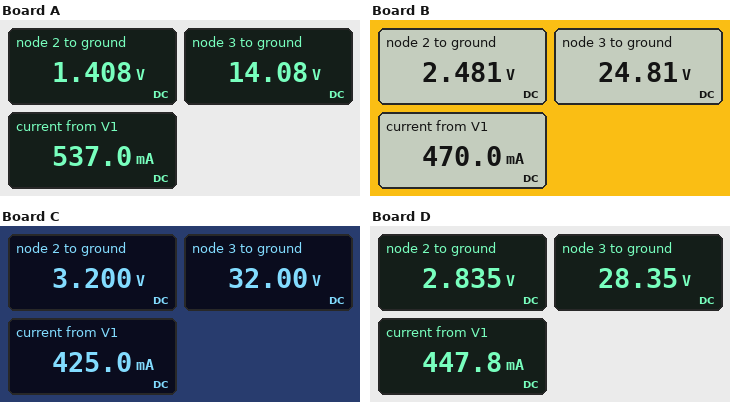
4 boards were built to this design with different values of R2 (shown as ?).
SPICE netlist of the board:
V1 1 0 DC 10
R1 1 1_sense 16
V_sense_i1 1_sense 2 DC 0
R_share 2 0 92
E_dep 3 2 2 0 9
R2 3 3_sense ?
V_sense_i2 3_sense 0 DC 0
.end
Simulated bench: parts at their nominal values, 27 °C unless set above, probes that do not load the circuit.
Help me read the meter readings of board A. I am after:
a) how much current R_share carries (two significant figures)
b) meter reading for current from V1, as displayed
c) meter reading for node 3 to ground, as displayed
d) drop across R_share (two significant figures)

15 mA
537.0 mA
14.08 V
1.4 V
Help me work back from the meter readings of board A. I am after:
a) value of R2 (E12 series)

27 Ω
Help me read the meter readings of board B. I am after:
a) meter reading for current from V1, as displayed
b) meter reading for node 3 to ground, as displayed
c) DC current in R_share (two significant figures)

470.0 mA
24.81 V
27 mA
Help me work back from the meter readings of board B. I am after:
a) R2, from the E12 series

56 Ω
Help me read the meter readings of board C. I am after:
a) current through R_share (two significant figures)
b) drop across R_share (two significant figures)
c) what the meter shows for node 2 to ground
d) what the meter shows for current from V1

35 mA
3.2 V
3.200 V
425.0 mA
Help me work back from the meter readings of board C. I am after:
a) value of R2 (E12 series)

82 Ω
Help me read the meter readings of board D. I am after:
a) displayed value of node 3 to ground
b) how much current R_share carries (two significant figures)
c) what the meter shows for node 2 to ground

28.35 V
31 mA
2.835 V
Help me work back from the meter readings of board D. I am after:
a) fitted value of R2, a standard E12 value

68 Ω
